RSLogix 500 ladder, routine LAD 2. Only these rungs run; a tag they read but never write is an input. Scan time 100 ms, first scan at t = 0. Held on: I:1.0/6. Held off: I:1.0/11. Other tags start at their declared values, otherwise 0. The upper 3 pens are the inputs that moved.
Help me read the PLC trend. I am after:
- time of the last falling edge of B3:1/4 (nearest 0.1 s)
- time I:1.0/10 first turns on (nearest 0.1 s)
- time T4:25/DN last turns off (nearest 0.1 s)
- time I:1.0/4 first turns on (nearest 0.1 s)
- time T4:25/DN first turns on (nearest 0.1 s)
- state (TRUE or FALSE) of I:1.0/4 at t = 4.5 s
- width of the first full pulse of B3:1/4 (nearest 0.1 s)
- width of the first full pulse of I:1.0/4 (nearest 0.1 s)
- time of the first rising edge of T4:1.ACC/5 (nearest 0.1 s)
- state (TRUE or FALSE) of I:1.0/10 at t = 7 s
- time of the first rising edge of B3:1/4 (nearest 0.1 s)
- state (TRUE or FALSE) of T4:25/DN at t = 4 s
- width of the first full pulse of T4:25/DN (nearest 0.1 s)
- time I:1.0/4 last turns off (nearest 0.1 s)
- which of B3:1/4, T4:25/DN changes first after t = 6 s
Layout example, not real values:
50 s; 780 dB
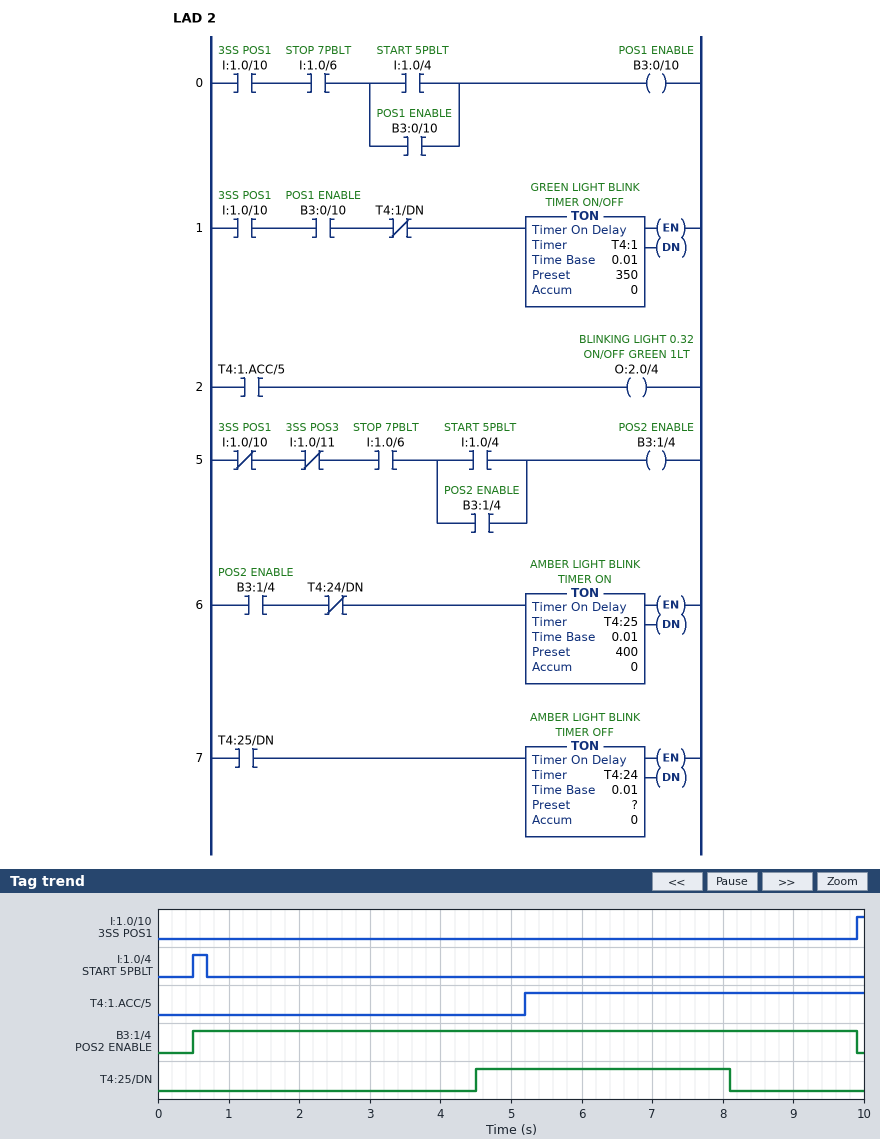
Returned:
9.9 s; 9.9 s; 8.1 s; 0.5 s; 4.5 s; FALSE; 9.4 s; 0.2 s; 5.2 s; FALSE; 0.5 s; FALSE; 3.6 s; 0.7 s; T4:25/DN
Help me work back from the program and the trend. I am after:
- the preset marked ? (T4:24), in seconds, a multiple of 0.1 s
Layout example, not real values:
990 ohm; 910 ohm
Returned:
3.5 s
